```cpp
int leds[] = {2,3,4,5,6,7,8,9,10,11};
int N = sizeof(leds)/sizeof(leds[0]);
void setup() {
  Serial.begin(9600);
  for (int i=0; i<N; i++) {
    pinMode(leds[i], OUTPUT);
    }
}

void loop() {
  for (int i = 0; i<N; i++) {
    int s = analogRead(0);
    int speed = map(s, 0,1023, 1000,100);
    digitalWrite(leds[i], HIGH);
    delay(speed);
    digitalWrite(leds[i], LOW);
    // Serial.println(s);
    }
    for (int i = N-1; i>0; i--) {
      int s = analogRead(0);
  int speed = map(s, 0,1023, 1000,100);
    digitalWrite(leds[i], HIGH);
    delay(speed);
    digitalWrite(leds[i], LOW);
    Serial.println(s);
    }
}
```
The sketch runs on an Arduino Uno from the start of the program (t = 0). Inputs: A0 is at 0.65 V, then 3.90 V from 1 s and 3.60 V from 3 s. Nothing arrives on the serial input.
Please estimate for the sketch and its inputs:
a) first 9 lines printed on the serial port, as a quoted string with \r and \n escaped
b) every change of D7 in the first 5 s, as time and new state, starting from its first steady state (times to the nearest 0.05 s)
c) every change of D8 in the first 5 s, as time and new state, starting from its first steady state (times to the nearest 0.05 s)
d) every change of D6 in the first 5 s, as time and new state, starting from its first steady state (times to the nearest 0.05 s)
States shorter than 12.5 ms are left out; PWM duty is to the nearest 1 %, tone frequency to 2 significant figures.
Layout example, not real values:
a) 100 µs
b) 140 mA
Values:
a) "737\r\n737\r\n737\r\n737\r\n737\r\n737\r\n737\r\n737\r\n737\r\n"
b) 0 s low; 2.65 s high; 2.95 s low
c) 0 s low; 2.95 s high; 3.25 s low
d) 0 s low; 2.35 s high; 2.65 s low
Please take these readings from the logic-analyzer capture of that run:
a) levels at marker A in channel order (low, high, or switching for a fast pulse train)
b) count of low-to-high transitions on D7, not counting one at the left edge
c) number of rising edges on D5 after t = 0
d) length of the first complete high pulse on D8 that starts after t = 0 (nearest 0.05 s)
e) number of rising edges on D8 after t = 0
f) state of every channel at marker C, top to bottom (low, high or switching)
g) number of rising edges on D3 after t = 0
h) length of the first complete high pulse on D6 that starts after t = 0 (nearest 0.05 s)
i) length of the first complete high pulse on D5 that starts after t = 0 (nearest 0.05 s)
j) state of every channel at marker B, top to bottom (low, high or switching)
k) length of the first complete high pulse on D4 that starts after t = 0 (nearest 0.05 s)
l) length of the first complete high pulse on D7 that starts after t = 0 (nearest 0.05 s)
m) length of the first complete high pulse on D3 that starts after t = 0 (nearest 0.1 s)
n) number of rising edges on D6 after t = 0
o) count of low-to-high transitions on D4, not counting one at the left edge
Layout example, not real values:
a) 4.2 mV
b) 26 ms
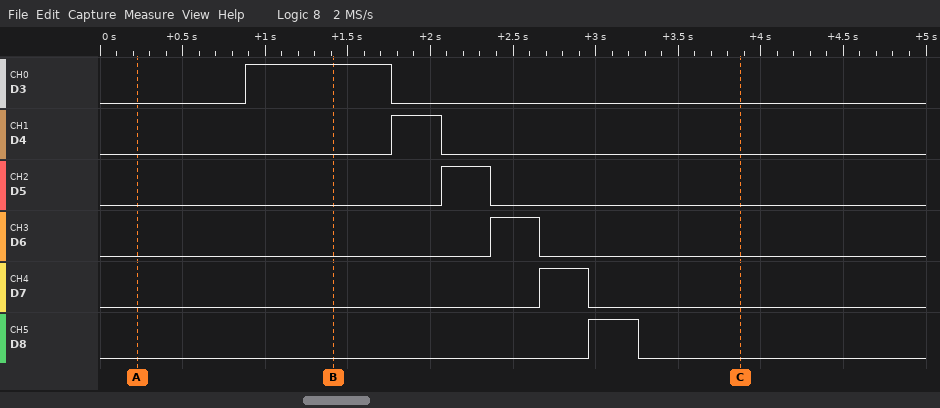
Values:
a) D3 low, D4 low, D5 low, D6 low, D7 low, D8 low
b) 1
c) 1
d) 0.30 s
e) 1
f) D3 low, D4 low, D5 low, D6 low, D7 low, D8 low
g) 1
h) 0.30 s
i) 0.30 s
j) D3 high, D4 low, D5 low, D6 low, D7 low, D8 low
k) 0.30 s
l) 0.30 s
m) 0.9 s
n) 1
o) 1
